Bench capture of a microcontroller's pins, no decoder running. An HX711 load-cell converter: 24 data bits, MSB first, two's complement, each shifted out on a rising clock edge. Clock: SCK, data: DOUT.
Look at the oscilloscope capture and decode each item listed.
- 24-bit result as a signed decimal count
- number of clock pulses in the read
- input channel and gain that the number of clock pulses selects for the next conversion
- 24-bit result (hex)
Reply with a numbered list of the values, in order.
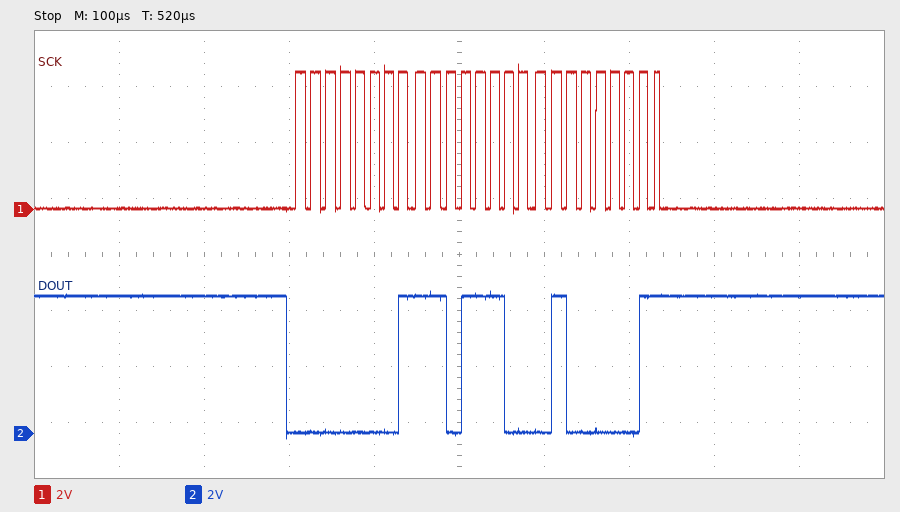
1. 121921
2. 25
3. channel A, gain 128
4. 0x01DC41
